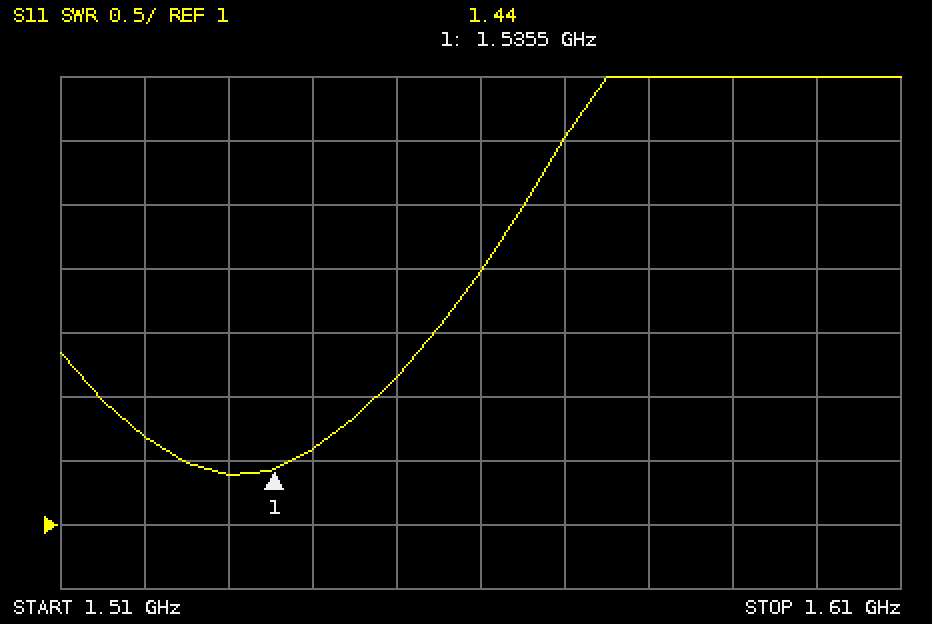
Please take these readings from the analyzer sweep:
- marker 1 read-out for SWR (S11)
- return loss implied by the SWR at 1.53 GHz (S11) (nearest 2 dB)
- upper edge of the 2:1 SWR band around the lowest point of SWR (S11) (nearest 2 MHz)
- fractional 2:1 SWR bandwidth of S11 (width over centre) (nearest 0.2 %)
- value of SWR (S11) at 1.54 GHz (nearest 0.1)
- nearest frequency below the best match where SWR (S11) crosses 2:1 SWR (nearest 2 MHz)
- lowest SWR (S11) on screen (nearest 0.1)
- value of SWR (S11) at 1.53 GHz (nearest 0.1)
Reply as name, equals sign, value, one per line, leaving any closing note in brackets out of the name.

marker 1 read-out for SWR = 1.44
return loss implied by the SWR at 1.53 GHz (S11) = 16 dB
upper edge of the 2:1 SWR band around the lowest point of SWR (S11) = 1.548 GHz
fractional 2:1 SWR bandwidth of S11 (width over centre) = 2.2 %
value of SWR (S11) at 1.54 GHz = 1.6
nearest frequency below the best match where SWR (S11) crosses 2:1 SWR = 1.514 GHz
lowest SWR (S11) on screen = 1.4
value of SWR (S11) at 1.53 GHz = 1.4
